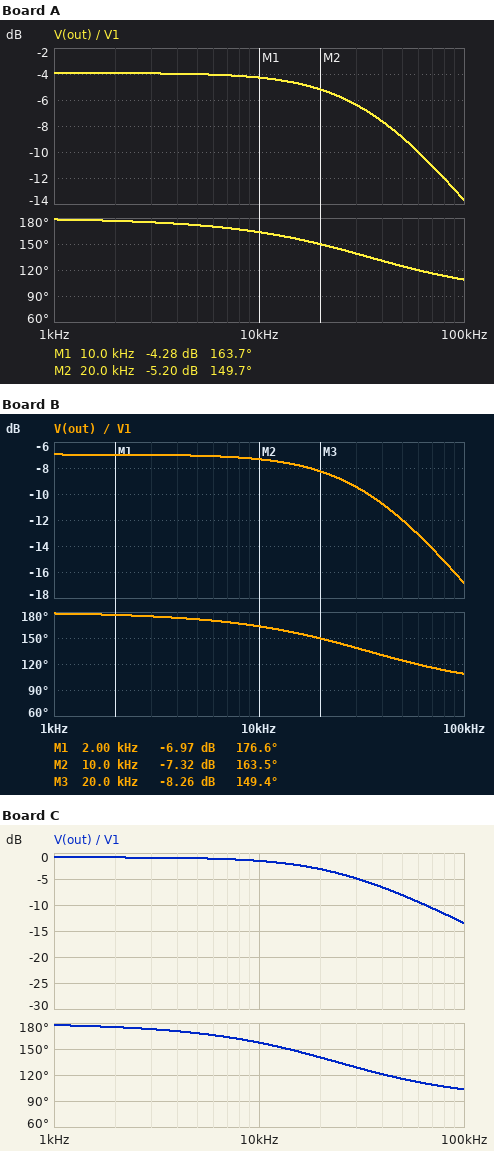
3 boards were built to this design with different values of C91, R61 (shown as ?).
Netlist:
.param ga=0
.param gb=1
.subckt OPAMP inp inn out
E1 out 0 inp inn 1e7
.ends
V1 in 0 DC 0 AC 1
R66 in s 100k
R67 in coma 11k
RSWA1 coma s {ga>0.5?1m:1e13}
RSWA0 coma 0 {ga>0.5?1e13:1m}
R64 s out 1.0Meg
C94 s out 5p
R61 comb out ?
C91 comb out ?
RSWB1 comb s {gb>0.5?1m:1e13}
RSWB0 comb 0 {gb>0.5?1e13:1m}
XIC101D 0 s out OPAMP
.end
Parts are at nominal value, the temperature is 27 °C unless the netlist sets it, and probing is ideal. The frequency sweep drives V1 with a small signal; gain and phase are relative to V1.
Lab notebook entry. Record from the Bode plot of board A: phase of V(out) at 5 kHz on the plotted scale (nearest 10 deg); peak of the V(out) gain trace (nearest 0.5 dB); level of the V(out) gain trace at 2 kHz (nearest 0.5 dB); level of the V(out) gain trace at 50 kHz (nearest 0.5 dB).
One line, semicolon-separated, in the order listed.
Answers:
170 deg; -4.0 dB; -4.0 dB; -9.0 dB
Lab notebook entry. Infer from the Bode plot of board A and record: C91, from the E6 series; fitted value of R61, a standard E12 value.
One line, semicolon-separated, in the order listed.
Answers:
68 pF; 68 kΩ
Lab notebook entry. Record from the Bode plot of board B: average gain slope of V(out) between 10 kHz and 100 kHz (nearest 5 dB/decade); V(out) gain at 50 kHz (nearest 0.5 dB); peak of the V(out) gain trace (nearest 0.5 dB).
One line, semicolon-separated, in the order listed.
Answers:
-10 dB/decade; -12.0 dB; -7.0 dB
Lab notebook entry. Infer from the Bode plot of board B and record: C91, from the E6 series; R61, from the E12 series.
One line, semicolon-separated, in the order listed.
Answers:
100 pF; 47 kΩ
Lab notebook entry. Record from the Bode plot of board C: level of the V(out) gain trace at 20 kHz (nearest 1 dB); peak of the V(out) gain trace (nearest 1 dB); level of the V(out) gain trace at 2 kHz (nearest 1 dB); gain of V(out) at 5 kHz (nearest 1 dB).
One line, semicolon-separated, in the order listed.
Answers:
-3 dB; -1 dB; -1 dB; -1 dB
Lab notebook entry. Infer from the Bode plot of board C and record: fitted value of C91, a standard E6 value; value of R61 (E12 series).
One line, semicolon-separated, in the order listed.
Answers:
68 pF; 100 kΩ
